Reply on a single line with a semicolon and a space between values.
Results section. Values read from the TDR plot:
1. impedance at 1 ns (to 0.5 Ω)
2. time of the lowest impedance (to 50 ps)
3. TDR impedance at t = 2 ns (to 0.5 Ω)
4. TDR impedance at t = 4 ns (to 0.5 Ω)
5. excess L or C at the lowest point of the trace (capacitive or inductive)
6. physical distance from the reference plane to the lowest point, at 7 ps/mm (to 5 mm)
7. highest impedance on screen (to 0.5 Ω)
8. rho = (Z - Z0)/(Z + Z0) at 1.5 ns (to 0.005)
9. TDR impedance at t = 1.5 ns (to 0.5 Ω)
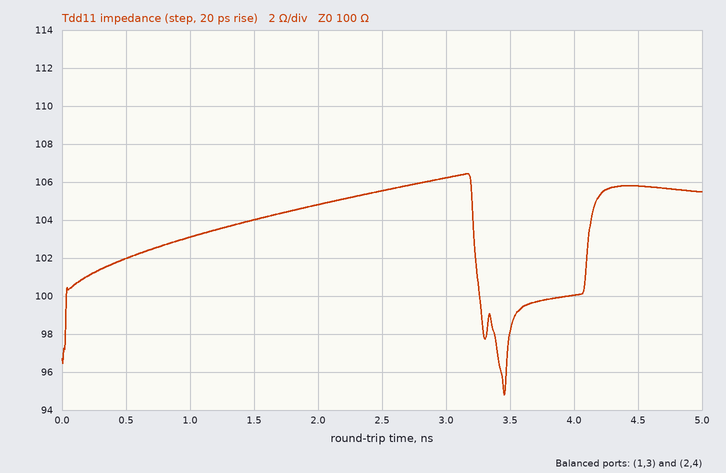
103.0 Ω; 3.45 ns; 105.0 Ω; 100.0 Ω; capacitive; 245 mm; 106.5 Ω; +0.020; 104.0 Ω
